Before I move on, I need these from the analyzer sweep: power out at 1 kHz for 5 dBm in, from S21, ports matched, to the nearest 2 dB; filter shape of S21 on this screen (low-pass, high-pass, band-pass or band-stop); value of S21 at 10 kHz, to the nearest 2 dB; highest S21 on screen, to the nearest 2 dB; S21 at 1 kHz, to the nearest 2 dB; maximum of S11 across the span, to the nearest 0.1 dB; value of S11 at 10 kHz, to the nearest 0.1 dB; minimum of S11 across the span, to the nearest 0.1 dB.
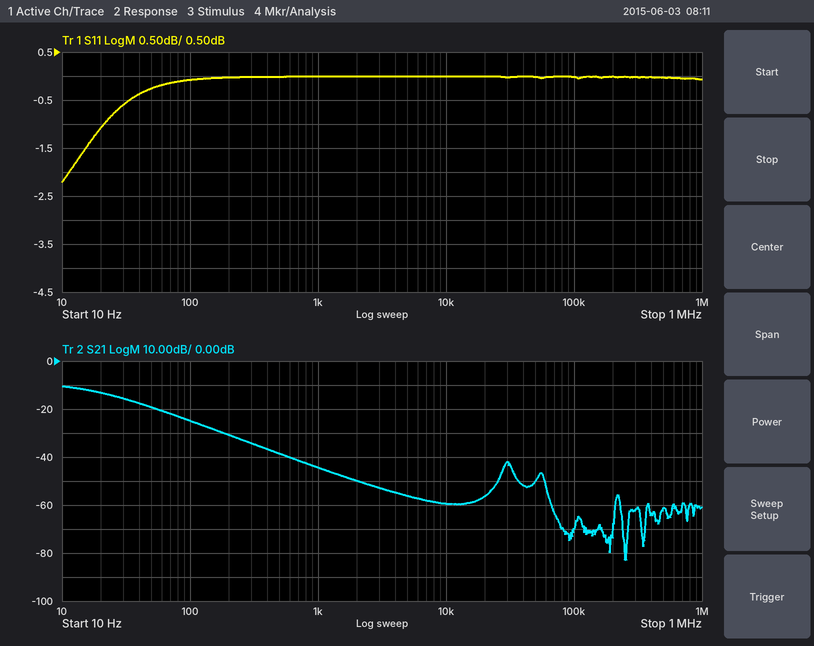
-40 dBm
low-pass
-60 dB
-10 dB
-44 dB
0.0 dB
0.0 dB
-2.2 dB
